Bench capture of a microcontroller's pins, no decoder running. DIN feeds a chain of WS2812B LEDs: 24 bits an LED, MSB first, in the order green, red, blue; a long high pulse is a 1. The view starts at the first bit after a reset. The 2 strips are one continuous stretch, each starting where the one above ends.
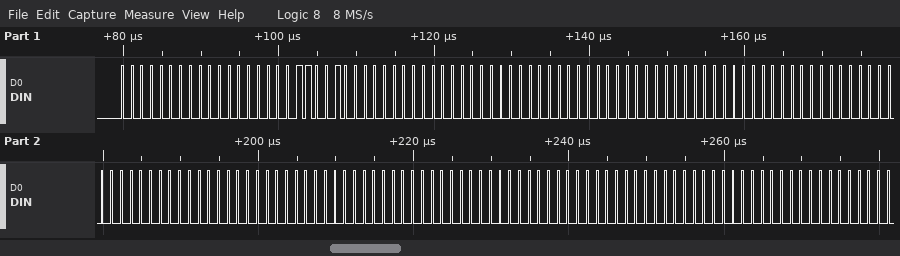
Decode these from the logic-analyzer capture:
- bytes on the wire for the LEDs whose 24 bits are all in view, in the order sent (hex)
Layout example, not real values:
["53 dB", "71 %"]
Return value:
["00 00 32 00 00 00 00 00 00 00 00 00 00 00 00 00 00 00"]
